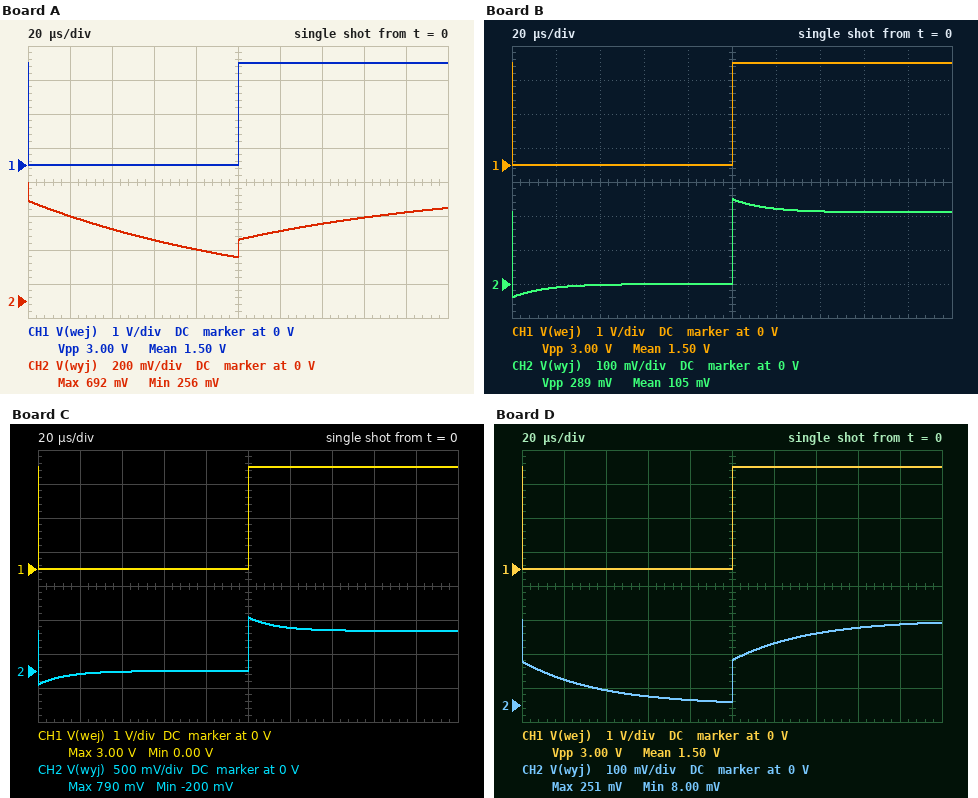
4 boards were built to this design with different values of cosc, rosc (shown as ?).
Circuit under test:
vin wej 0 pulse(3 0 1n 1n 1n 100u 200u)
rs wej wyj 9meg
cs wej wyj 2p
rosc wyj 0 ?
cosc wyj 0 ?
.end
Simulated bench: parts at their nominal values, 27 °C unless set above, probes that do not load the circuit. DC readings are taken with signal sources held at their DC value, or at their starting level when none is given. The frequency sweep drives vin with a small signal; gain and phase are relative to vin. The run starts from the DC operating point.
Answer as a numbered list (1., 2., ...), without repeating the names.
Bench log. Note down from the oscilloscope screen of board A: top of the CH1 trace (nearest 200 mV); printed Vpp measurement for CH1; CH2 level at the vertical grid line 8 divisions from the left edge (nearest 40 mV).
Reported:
1. 3.0 V
2. 3.00 V
3. 480 mV
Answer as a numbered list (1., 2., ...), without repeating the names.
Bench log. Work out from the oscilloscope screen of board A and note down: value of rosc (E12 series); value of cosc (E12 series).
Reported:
1. 2.7 MΩ
2. 56 pF
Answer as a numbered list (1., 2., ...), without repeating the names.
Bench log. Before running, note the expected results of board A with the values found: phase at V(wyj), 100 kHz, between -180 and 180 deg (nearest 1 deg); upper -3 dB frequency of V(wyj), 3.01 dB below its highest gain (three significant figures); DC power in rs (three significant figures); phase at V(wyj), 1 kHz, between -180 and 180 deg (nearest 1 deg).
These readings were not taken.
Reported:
1. -4 deg
2. 1.35 kHz
3. 592 nW
4. -31 deg
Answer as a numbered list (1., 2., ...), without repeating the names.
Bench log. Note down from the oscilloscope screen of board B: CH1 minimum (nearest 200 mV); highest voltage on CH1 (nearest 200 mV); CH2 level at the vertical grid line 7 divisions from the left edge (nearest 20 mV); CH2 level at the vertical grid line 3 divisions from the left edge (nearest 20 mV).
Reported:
1. 0 V
2. 3.0 V
3. 220 mV
4. 0 V
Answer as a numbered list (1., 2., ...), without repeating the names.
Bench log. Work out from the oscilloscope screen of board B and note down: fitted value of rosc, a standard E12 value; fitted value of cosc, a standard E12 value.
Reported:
1. 680 kΩ
2. 22 pF
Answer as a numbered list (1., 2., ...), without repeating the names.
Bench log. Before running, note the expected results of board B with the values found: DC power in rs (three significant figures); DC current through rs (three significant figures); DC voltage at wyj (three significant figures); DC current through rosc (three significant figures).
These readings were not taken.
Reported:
1. 864 nW
2. 310 nA
3. 211 mV
4. 310 nA
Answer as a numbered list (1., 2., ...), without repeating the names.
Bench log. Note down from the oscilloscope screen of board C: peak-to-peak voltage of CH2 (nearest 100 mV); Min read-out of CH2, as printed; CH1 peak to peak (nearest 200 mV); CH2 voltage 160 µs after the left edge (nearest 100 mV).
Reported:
1. 1.0 V
2. -200 mV
3. 3.0 V
4. 600 mV
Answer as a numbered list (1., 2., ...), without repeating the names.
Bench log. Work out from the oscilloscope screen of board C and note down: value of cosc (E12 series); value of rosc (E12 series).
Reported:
1. 5.6 pF
2. 2.2 MΩ
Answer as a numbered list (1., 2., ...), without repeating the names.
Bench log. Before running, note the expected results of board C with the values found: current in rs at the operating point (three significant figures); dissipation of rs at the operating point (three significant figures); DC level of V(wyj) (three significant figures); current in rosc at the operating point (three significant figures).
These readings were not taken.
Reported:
1. 268 nA
2. 646 nW
3. 589 mV
4. 268 nA
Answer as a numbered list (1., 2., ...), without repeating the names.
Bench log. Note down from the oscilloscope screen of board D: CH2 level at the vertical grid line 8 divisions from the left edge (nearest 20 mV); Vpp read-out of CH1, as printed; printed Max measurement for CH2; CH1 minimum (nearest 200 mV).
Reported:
1. 220 mV
2. 3.00 V
3. 251 mV
4. 0 V
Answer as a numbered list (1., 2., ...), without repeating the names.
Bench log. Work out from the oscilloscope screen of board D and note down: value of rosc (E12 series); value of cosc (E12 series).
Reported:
1. 820 kΩ
2. 47 pF
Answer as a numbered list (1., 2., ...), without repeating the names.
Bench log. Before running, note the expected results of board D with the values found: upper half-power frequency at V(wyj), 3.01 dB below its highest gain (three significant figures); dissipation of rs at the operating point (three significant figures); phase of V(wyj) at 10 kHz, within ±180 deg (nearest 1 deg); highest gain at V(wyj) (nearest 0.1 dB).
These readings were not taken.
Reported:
1. 5.98 kHz
2. 840 nW
3. -18 deg
4. -21.6 dB
